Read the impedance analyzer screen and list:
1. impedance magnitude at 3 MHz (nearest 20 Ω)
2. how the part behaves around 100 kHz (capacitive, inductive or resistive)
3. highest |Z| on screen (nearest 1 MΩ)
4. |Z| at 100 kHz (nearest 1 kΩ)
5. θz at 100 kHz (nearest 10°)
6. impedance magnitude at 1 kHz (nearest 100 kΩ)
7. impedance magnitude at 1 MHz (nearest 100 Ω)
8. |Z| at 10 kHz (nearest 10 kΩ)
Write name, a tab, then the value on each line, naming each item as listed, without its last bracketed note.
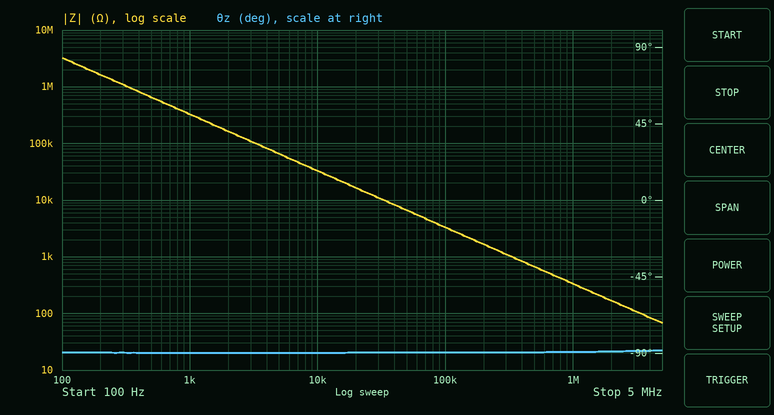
impedance magnitude at 3 MHz	120 Ω
how the part behaves around 100 kHz	capacitive
highest |Z| on screen	3 MΩ
|Z| at 100 kHz	3 kΩ
θz at 100 kHz	-90°
impedance magnitude at 1 kHz	300 kΩ
impedance magnitude at 1 MHz	300 Ω
|Z| at 10 kHz	30 kΩ
